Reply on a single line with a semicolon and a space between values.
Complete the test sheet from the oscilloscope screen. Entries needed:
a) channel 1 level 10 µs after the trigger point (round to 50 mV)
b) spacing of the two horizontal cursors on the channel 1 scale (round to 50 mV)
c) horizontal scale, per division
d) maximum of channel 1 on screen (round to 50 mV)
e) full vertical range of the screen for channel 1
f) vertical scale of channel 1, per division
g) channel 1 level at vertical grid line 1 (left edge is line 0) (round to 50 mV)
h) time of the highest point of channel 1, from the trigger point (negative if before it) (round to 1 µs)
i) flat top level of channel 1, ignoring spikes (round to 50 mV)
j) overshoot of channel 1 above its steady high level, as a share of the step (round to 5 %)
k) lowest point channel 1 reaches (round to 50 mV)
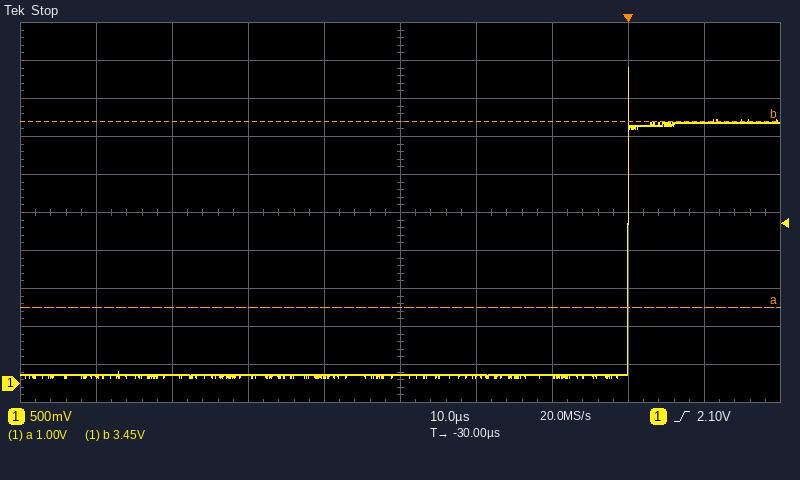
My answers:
3.45 V; 2.45 V; 10 µs; 4.15 V; 5 V; 500 mV; 100 mV; 0 µs; 3.45 V; 20 %; 100 mV
